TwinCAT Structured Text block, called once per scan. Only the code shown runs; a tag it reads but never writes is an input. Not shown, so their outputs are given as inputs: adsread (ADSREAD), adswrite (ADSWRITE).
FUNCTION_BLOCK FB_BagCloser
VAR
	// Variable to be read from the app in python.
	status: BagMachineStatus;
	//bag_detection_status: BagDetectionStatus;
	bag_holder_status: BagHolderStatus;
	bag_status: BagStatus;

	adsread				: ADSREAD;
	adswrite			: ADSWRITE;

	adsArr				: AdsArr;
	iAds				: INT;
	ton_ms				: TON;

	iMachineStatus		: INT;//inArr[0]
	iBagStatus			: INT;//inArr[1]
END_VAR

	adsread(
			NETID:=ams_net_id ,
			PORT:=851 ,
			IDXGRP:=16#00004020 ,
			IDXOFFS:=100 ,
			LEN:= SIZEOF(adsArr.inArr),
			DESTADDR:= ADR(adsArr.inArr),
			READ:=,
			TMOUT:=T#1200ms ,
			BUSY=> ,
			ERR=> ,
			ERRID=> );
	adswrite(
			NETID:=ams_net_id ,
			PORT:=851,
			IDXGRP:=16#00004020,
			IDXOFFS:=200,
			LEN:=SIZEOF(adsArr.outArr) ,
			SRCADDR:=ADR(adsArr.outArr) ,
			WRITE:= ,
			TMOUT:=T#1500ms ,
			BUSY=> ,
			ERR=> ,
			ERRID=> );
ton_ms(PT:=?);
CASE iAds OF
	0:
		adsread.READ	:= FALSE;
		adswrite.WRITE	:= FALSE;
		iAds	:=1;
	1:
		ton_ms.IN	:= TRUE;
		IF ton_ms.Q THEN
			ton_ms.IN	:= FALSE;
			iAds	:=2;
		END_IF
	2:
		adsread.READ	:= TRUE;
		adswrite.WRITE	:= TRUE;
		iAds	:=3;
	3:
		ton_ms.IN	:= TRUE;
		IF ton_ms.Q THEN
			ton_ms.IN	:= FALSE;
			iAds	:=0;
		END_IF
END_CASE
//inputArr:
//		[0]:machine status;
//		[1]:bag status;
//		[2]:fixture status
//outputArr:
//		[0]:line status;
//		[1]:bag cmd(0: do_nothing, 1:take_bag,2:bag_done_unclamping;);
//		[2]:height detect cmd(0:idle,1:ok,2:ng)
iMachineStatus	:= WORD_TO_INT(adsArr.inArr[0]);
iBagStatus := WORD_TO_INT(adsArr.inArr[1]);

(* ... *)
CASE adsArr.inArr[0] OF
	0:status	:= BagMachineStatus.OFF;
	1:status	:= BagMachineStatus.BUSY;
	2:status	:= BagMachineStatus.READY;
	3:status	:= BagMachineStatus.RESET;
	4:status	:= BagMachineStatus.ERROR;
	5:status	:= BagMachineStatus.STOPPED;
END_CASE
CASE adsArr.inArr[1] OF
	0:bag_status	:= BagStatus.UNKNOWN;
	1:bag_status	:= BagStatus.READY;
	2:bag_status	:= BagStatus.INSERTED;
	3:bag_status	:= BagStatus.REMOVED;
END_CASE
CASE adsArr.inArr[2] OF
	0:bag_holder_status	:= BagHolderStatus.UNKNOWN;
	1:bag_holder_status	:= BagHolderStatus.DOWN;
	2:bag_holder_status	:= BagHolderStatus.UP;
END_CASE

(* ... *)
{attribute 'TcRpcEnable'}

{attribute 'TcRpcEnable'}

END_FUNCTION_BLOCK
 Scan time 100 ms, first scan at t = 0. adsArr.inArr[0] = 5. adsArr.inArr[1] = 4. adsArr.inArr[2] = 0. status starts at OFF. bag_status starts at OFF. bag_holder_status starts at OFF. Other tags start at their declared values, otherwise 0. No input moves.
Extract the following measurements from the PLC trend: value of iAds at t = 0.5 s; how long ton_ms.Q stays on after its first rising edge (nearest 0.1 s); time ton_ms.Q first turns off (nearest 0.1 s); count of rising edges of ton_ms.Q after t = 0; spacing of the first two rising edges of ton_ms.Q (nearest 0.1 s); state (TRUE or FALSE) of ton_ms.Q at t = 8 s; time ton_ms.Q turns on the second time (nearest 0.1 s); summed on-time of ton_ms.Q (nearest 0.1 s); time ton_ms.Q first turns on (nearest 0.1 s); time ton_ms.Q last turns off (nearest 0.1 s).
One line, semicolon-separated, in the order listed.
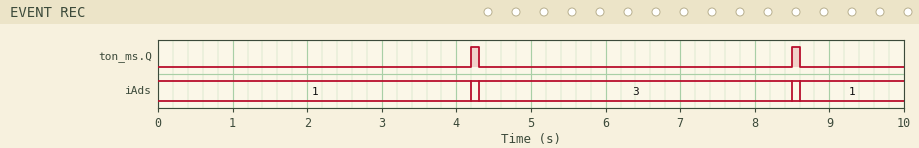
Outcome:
1; 0.1 s; 4.3 s; 2; 4.3 s; FALSE; 8.5 s; 0.2 s; 4.2 s; 8.6 s
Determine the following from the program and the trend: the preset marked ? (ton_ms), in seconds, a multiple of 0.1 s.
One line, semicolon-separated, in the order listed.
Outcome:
4.0 s
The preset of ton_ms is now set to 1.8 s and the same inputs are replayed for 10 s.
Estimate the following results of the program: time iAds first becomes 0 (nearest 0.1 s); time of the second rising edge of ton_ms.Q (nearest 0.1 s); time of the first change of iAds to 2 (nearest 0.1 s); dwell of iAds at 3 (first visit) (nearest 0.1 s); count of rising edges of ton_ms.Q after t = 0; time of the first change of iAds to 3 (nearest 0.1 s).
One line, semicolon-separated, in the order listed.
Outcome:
4.1 s; 4.1 s; 2.0 s; 2.0 s; 4; 2.1 s
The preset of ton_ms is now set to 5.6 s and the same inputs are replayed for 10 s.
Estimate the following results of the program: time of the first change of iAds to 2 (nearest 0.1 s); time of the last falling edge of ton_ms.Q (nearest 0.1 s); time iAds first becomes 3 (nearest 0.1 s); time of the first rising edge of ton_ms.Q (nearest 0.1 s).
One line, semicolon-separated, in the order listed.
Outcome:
5.8 s; 5.9 s; 5.9 s; 5.8 s
